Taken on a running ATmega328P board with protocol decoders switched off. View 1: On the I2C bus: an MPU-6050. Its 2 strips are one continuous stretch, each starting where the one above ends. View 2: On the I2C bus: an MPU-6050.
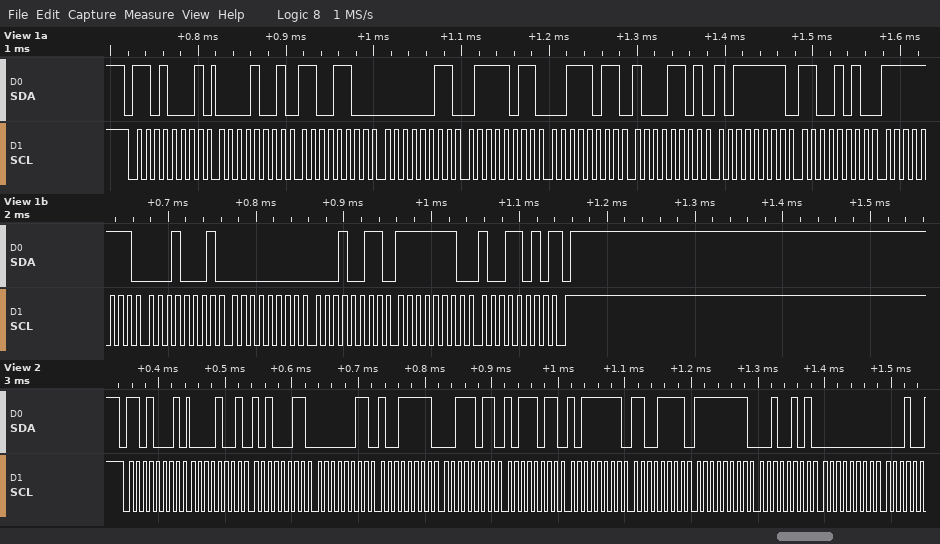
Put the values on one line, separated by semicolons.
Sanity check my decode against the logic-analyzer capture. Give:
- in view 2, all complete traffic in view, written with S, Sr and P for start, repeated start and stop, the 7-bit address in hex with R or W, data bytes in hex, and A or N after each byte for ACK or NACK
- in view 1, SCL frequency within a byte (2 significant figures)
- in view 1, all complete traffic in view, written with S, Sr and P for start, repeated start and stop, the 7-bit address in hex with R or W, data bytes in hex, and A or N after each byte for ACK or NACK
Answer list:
S 68R A 09 A A3 A 03 A 9F A 3B A BB A BF A CF A FF A 25 A 00 A; 100 kHz; S 68R A 09 A CC A 03 A 7B A 3B A 8D A BF A CA A FF A 11 A 00 A 13 A FE A 9A N P
